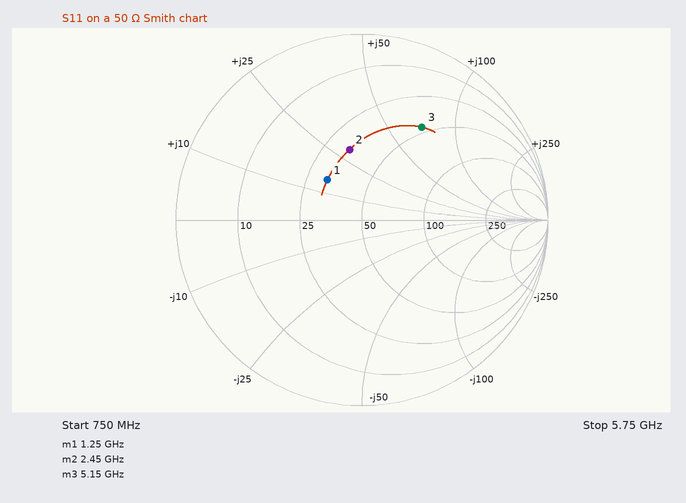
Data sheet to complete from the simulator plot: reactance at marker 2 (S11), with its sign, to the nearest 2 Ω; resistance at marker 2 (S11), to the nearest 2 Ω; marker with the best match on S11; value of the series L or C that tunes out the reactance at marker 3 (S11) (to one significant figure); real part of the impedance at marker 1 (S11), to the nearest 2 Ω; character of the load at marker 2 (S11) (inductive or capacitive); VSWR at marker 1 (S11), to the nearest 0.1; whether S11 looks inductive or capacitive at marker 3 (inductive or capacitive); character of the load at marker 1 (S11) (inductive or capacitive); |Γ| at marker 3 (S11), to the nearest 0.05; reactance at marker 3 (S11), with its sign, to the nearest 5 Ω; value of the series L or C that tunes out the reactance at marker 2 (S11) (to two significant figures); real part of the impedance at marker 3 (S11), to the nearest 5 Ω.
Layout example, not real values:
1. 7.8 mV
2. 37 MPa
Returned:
1. +30 Ω
2. 34 Ω
3. marker 1
4. 400 fF
5. 32 Ω
6. inductive
7. 1.8
8. inductive
9. inductive
10. 0.60
11. +70 Ω
12. 2.2 pF
13. 45 Ω
